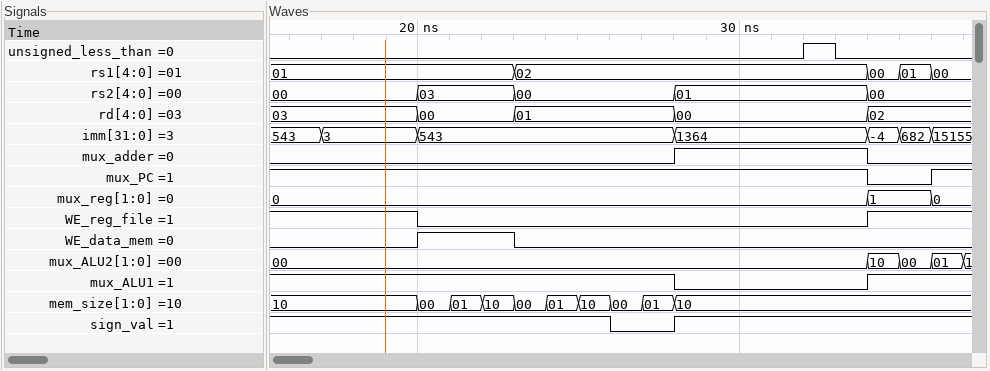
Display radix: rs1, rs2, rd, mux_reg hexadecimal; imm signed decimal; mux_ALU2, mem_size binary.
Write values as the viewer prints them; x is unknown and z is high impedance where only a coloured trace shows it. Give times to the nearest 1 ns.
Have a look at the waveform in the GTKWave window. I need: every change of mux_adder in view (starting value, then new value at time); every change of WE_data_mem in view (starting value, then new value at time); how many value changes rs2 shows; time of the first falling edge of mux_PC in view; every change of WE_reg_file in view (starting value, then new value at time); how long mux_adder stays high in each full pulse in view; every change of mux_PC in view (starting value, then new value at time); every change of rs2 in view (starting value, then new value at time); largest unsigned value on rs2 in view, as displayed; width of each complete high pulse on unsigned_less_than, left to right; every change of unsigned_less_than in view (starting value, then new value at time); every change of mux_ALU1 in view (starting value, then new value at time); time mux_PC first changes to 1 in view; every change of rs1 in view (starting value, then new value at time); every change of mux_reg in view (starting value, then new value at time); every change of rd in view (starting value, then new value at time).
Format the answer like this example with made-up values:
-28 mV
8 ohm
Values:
0, 1 at 28 ns, 0 at 34 ns
0, 1 at 20 ns, 0 at 23 ns
4
34 ns
1, 0 at 20 ns, 1 at 34 ns
6 ns
1, 0 at 34 ns, 1 at 36 ns
00, 03 at 20 ns, 00 at 23 ns, 01 at 28 ns, 00 at 34 ns
03
1 ns
0, 1 at 32 ns, 0 at 33 ns
1, 0 at 28 ns, 1 at 34 ns
36 ns
01, 02 at 23 ns, 00 at 34 ns, 01 at 35 ns, 00 at 36 ns
0, 1 at 34 ns, 0 at 36 ns
03, 00 at 20 ns, 01 at 23 ns, 00 at 28 ns, 02 at 34 ns
